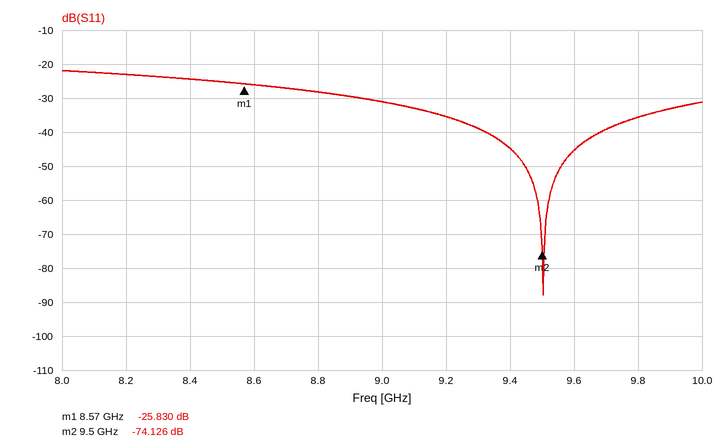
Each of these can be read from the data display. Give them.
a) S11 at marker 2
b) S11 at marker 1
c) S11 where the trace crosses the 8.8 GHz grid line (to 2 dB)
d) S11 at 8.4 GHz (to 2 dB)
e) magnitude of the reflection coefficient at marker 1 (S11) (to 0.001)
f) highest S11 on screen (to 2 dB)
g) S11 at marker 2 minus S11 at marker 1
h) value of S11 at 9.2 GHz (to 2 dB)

-74.126 dB
-25.830 dB
-28 dB
-24 dB
0.051
-22 dB
-48.296 dB
-36 dB
